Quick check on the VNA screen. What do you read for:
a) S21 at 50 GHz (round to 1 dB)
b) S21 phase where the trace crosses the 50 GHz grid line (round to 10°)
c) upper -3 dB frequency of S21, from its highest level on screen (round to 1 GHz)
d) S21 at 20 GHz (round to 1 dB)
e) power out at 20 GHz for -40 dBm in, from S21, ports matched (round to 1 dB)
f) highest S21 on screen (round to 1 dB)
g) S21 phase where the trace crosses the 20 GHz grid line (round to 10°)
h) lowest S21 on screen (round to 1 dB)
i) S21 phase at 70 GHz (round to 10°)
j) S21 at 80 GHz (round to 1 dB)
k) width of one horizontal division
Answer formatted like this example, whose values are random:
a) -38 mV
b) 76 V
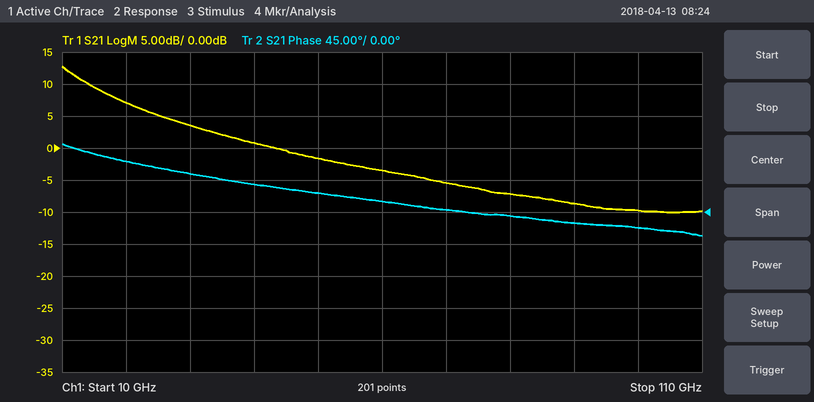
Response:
a) -2 dB
b) 30°
c) 15 GHz
d) 7 dB
e) -33 dBm
f) 13 dB
g) 70°
h) -10 dB
i) 0°
j) -7 dB
k) 10 GHz
